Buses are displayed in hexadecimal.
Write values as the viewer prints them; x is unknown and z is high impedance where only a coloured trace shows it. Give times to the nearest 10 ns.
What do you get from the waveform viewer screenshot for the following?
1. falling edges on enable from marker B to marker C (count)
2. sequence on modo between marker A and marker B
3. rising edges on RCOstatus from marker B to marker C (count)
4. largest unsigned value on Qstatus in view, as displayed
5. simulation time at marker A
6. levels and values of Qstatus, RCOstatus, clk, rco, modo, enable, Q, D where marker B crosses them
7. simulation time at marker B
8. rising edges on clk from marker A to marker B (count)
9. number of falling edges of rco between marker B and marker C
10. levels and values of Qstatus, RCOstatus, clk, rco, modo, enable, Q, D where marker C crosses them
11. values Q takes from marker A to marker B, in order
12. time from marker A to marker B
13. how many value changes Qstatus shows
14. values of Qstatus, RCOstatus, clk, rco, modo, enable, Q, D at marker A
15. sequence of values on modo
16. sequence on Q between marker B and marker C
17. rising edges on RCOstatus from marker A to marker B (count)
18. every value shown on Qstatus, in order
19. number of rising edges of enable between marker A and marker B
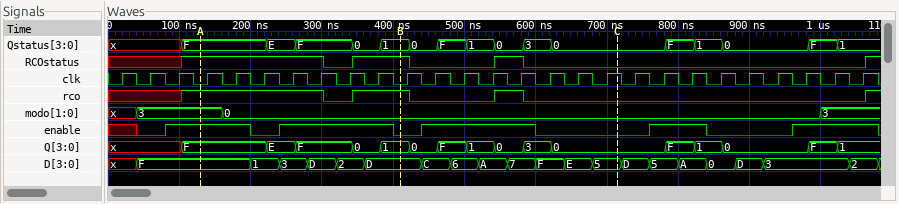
1
3, 0
1
F
130 ns
Qstatus=1, RCOstatus=1, clk=0, rco=1, modo=0, enable=0, Q=1, D=D
410 ns
7
2
Qstatus=0, RCOstatus=0, clk=1, rco=0, modo=0, enable=0, Q=0, D=5
F, E, F, 0, 1
280 ns
16
Qstatus=F, RCOstatus=1, clk=0, rco=1, modo=3, enable=1, Q=F, D=F
x, 3, 0, 3
1, 0, F, 1, 0, 3, 0
1
x, F, E, F, 0, 1, 0, F, 1, 0, 3, 0, F, 1, 0, F, 1
1
